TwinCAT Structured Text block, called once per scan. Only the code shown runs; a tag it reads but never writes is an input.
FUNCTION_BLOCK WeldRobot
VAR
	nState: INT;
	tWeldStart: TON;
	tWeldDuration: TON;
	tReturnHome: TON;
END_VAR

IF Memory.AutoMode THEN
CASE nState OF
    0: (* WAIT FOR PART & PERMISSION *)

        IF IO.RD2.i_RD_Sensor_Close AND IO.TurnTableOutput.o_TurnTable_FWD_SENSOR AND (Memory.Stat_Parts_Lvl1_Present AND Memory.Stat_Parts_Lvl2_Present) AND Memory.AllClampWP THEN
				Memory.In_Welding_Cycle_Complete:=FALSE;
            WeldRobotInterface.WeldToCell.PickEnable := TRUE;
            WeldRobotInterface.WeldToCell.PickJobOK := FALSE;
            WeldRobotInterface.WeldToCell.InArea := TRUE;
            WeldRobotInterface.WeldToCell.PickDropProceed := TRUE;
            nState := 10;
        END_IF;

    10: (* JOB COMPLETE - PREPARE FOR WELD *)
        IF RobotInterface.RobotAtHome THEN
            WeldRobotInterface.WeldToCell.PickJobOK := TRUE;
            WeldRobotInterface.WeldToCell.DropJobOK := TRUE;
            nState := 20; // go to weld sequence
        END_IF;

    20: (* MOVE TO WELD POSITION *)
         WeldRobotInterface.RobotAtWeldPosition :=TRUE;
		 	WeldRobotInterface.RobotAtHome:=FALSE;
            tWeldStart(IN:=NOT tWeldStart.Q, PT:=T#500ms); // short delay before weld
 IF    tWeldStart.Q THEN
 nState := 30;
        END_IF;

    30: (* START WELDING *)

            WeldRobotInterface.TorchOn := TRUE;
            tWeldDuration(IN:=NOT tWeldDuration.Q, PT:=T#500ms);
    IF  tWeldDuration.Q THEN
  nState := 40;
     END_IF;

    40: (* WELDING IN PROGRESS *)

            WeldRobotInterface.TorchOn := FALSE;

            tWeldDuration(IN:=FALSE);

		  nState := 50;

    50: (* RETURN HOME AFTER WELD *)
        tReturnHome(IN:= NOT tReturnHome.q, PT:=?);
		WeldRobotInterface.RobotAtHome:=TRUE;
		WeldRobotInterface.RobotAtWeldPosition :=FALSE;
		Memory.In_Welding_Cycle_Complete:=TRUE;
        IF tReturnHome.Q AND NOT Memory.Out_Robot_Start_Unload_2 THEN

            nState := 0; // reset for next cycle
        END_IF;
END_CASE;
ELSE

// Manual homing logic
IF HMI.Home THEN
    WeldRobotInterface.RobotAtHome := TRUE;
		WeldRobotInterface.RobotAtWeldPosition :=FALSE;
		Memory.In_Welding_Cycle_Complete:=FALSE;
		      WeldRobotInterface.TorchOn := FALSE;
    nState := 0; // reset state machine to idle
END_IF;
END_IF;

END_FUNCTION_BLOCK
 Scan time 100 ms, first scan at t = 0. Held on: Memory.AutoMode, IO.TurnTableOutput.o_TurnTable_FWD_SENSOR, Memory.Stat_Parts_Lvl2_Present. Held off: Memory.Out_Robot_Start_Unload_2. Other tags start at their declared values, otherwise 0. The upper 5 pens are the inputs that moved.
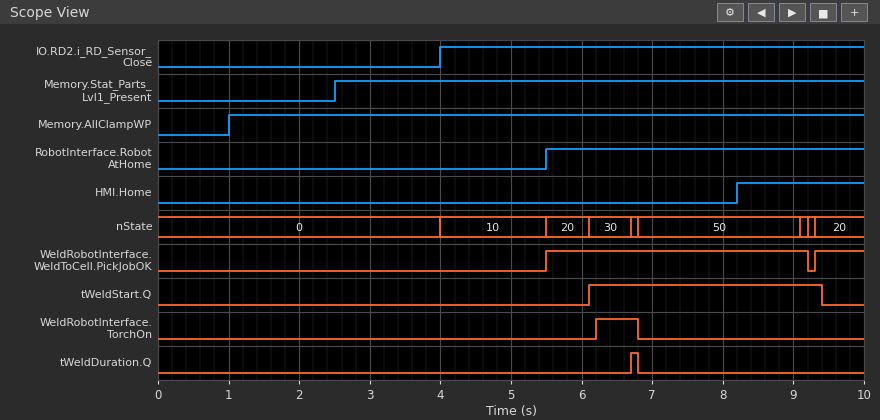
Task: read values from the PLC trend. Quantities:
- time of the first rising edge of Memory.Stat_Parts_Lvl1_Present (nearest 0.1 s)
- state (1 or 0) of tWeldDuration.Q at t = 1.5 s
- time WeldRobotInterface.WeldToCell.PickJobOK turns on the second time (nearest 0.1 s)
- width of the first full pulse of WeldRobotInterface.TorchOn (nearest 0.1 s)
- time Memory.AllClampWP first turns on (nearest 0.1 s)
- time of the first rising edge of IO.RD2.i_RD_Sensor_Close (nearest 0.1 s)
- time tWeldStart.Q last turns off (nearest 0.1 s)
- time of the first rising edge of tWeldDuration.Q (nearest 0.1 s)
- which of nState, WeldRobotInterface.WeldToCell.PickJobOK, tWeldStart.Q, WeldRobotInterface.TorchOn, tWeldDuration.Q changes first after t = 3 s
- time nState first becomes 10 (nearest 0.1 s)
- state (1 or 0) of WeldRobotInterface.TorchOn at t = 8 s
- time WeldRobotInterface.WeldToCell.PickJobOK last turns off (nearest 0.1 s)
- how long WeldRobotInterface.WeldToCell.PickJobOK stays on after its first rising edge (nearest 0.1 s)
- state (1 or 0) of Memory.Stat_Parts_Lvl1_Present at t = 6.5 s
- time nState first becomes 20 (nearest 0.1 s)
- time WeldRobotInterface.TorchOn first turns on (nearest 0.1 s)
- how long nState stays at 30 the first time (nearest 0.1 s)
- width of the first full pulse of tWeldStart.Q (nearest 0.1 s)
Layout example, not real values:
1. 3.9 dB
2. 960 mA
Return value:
1. 2.5 s
2. 0
3. 9.3 s
4. 0.6 s
5. 1.0 s
6. 4.0 s
7. 9.4 s
8. 6.7 s
9. nState
10. 4.0 s
11. 0
12. 9.2 s
13. 3.7 s
14. 1
15. 5.5 s
16. 6.2 s
17. 0.6 s
18. 3.3 s
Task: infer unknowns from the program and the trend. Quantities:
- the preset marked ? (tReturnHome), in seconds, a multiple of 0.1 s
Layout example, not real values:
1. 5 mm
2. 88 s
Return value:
1. 2.2 s
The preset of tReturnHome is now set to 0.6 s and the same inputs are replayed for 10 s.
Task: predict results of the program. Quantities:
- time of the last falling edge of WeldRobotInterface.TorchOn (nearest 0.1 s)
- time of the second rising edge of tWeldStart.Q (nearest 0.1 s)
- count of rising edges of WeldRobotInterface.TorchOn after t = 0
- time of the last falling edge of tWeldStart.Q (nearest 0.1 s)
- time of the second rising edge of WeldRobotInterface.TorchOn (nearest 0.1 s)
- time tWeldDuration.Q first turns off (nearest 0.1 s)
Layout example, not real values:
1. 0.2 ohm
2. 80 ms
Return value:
1. 9.1 s
2. 8.4 s
3. 2
4. 7.8 s
5. 8.5 s
6. 6.8 s
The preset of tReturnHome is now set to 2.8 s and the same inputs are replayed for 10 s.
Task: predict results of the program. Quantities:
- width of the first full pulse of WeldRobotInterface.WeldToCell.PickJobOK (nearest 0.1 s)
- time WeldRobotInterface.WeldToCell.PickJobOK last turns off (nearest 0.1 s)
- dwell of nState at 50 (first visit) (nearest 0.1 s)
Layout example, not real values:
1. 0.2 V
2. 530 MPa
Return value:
1. 4.3 s
2. 9.8 s
3. 2.9 s
